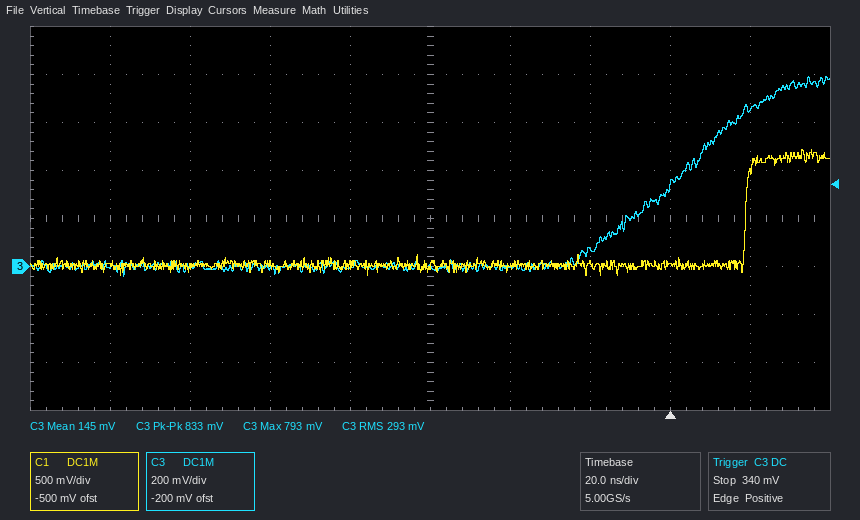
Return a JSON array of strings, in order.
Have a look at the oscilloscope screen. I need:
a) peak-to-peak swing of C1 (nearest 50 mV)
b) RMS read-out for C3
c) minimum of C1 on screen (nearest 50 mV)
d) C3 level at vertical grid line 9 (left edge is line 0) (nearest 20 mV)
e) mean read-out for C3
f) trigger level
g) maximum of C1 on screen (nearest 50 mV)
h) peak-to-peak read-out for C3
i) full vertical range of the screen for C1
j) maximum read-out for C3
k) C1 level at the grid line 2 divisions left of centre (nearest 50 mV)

["1.30 V", "293 mV", "-100 mV", "660 mV", "145 mV", "340 mV", "1.20 V", "833 mV", "4 V", "793 mV", "0 mV"]
